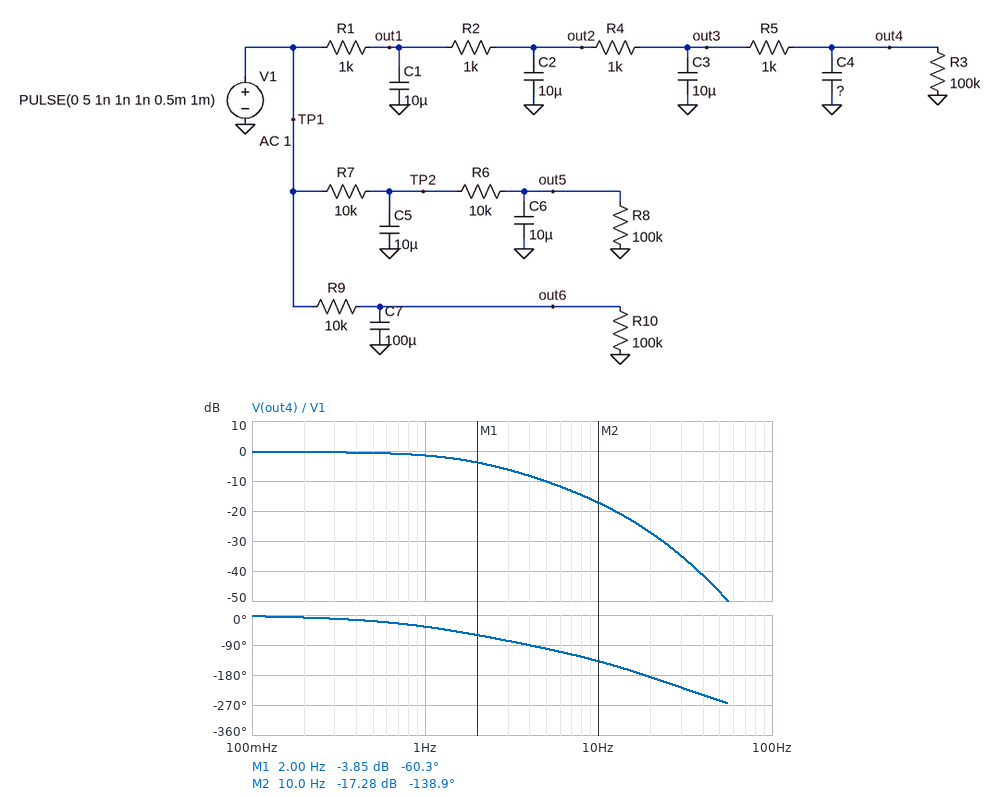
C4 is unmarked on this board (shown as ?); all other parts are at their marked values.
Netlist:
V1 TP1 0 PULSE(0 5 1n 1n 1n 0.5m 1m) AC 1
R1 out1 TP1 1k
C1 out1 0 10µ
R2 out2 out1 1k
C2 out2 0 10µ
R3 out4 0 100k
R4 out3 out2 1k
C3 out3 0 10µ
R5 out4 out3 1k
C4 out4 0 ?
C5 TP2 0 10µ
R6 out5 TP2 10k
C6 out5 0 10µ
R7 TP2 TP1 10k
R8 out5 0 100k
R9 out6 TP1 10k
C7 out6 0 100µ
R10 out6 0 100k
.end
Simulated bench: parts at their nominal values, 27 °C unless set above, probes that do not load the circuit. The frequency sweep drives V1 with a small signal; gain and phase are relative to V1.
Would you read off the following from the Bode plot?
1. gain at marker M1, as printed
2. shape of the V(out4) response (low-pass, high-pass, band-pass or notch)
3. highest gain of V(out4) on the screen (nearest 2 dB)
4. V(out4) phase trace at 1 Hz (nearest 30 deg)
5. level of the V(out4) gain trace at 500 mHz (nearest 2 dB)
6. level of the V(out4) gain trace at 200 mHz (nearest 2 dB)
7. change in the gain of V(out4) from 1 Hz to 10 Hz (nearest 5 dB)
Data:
-3.85 dB
low-pass
0 dB
-30 deg
0 dB
0 dB
-15 dB
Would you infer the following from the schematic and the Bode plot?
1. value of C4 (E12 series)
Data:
12 µF
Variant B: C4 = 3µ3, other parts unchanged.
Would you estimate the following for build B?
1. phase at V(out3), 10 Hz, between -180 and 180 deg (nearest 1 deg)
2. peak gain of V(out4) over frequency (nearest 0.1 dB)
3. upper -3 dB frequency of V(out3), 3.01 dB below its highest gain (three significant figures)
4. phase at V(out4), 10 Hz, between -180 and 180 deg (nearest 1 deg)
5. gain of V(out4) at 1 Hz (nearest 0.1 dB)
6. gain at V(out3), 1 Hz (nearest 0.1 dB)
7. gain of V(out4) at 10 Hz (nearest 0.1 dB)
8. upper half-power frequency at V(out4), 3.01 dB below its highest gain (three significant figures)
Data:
-108 deg
-0.3 dB
2.68 Hz
-119 deg
-0.9 dB
-0.8 dB
-13.1 dB
2.67 Hz
